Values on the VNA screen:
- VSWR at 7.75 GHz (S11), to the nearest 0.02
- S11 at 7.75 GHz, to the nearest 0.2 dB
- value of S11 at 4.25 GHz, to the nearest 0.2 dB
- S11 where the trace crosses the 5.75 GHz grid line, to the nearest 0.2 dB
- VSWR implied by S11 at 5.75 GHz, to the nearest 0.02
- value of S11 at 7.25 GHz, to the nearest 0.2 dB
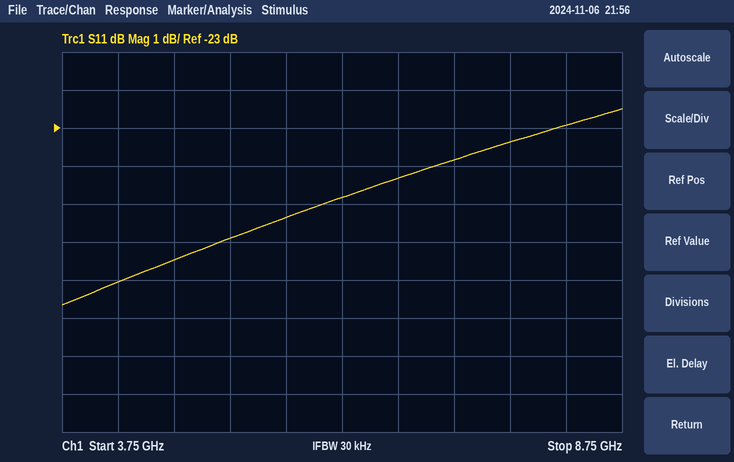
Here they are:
1.14
-23.4 dB
-27.0 dB
-25.4 dB
1.12
-23.8 dB
